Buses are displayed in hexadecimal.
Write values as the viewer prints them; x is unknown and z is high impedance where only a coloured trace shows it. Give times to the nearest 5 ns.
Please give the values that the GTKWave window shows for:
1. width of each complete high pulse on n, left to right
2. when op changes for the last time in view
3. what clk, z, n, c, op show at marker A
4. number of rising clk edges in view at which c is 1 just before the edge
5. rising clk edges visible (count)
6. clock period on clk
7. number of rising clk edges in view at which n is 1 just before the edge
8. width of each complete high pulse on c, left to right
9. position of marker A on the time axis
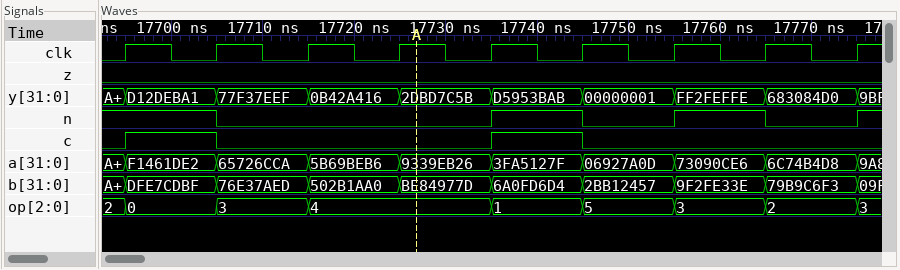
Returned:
10 ns, 10 ns
17775 ns
clk=1, z=0, n=0, c=0, op=4
2
9
10 ns
4
10 ns, 10 ns
17725 ns
